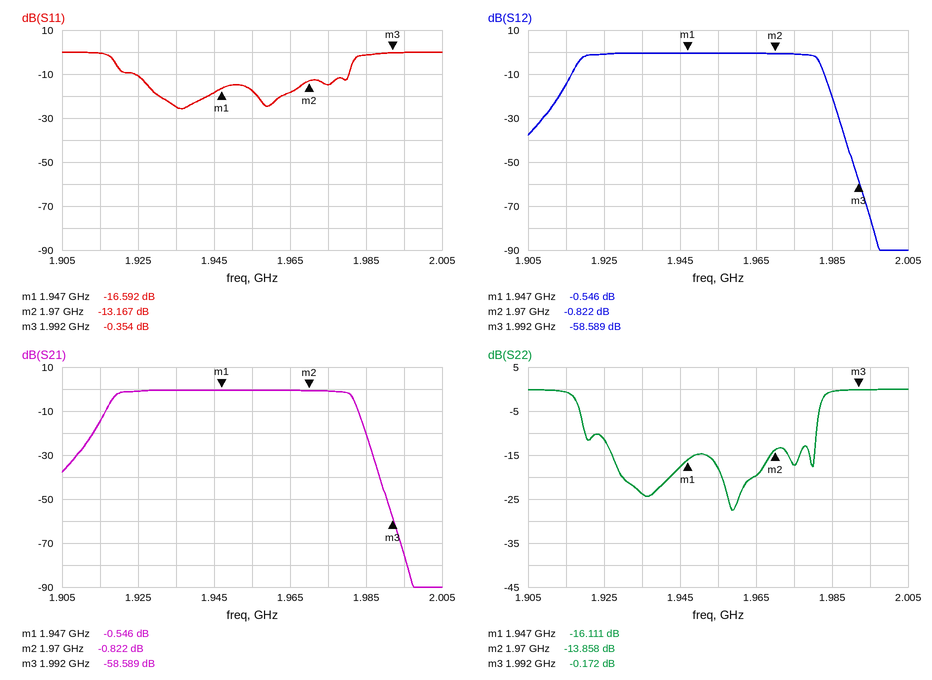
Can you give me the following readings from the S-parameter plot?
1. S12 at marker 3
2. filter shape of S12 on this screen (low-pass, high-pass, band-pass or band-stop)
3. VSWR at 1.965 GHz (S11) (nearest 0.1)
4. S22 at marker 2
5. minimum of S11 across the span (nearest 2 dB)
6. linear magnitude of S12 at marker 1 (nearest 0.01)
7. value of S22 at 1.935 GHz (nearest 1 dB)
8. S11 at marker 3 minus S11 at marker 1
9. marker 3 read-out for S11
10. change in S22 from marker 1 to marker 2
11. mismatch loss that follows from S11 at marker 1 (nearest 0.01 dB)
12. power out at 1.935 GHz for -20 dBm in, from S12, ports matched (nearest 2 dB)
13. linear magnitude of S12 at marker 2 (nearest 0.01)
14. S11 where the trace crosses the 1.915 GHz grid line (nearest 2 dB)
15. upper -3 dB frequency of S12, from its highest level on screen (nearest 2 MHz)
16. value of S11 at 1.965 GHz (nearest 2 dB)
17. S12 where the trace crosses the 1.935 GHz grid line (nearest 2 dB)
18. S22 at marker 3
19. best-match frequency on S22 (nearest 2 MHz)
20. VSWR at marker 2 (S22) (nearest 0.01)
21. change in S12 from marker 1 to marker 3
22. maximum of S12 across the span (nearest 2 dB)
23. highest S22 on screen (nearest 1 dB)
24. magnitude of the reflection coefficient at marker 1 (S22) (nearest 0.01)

-58.589 dB
band-pass
1.3
-13.858 dB
-26 dB
0.94
-24 dB
16.238 dB
-0.354 dB
2.253 dB
0.10 dB
-20 dBm
0.91
0 dB
1.982 GHz
-18 dB
0 dB
-0.172 dB
1.958 GHz
1.51
-58.043 dB
0 dB
0 dB
0.16
